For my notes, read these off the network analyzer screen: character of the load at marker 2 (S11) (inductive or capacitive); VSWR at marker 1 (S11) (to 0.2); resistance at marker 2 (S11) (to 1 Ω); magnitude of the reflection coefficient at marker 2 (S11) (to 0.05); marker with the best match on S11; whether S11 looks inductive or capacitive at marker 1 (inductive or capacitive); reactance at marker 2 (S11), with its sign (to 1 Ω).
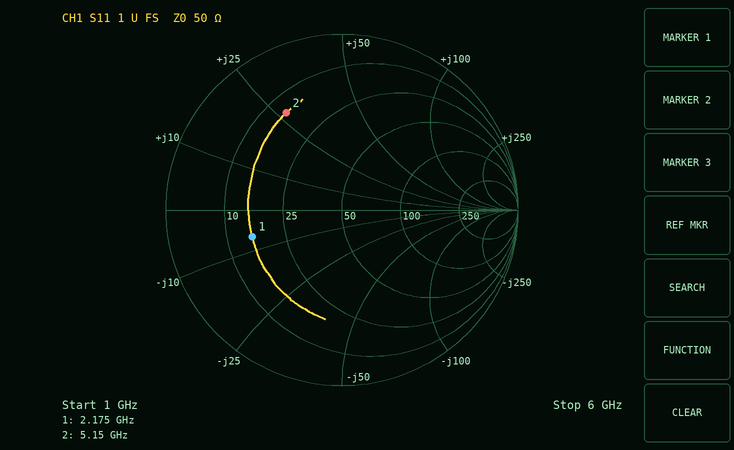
inductive
3.2
15 Ω
0.65
marker 1
capacitive
+27 Ω
